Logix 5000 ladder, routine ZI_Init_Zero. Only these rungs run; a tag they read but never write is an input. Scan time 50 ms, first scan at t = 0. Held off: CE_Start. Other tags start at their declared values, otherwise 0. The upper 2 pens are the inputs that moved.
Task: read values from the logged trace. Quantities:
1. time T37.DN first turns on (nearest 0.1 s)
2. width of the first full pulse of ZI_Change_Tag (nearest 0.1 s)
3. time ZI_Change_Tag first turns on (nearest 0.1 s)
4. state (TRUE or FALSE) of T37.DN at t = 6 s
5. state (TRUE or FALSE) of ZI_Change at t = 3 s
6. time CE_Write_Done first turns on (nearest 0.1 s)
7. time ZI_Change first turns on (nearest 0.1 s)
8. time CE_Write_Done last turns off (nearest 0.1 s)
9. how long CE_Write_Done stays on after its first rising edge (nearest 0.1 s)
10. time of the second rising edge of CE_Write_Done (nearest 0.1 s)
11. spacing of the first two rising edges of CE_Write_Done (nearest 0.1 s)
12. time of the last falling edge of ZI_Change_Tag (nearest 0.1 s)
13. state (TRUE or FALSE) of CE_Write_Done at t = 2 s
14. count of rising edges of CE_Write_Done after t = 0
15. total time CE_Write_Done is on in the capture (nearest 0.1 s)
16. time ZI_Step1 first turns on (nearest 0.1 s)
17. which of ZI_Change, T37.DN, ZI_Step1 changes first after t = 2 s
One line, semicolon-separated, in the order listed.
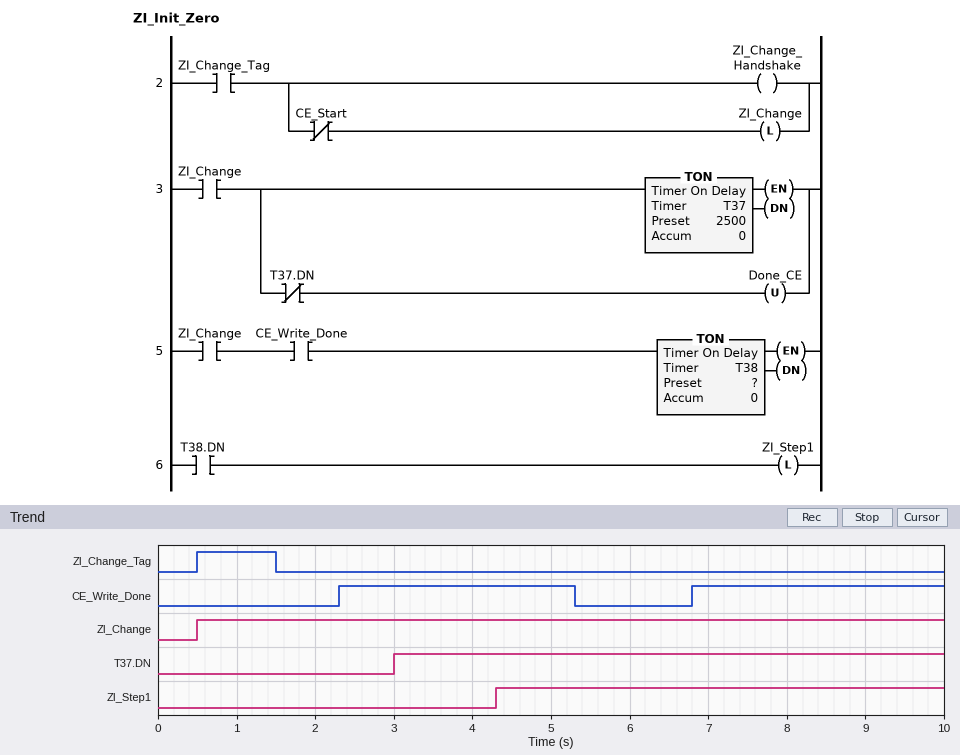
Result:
3.0 s; 1.0 s; 0.5 s; TRUE; TRUE; 2.3 s; 0.5 s; 5.3 s; 3.0 s; 6.8 s; 4.5 s; 1.5 s; FALSE; 2; 6.2 s; 4.3 s; T37.DN
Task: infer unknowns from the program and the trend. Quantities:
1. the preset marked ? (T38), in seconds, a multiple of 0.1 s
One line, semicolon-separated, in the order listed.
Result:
2.0 s
